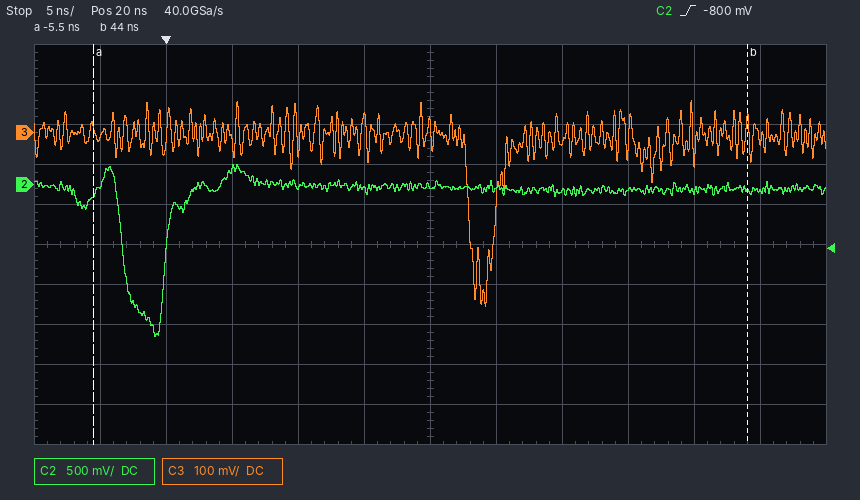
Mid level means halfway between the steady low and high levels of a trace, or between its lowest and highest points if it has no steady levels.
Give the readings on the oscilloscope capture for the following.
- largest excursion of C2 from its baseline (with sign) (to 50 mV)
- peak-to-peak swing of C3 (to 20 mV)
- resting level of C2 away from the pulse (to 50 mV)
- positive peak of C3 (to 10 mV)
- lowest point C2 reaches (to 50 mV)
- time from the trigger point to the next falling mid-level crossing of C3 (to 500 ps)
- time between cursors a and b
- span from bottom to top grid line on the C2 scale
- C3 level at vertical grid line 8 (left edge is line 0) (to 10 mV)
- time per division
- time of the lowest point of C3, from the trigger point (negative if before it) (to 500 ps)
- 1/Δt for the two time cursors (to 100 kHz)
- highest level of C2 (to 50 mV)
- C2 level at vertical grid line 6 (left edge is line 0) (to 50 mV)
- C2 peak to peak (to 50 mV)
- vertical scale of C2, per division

-1.85 V
520 mV
-50 mV
80 mV
-1.90 V
23.0 ns
49.5 ns
5 V
-20 mV
5 ns
+24.0 ns
20.2 MHz
250 mV
0 mV
2.15 V
500 mV
